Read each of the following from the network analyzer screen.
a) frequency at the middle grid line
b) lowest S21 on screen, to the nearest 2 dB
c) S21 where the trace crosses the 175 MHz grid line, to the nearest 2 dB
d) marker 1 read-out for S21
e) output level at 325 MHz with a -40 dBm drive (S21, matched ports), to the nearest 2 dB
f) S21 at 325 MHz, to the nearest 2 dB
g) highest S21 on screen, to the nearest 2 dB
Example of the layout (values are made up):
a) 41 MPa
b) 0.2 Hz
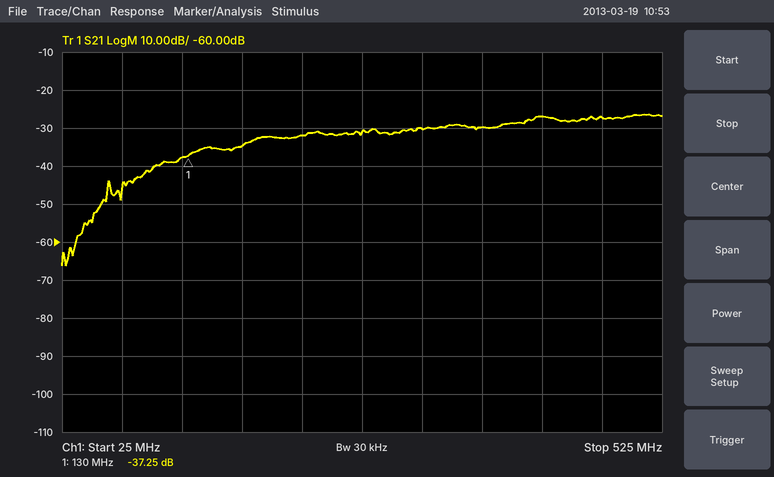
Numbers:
a) 275 MHz
b) -66 dB
c) -34 dB
d) -37.25 dB
e) -70 dBm
f) -30 dB
g) -26 dB
